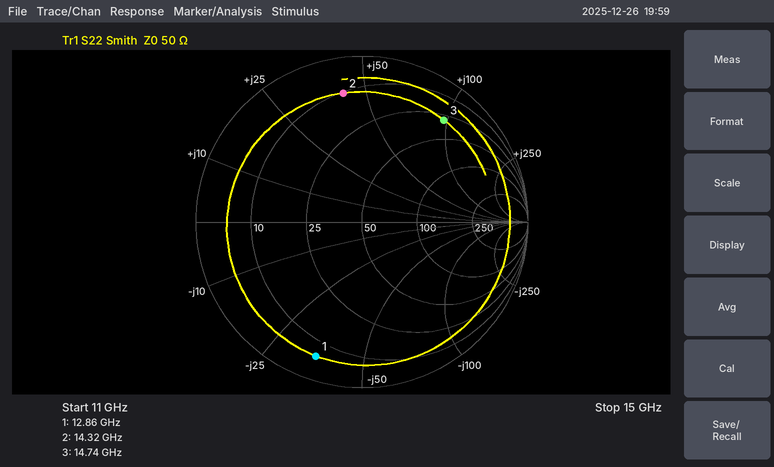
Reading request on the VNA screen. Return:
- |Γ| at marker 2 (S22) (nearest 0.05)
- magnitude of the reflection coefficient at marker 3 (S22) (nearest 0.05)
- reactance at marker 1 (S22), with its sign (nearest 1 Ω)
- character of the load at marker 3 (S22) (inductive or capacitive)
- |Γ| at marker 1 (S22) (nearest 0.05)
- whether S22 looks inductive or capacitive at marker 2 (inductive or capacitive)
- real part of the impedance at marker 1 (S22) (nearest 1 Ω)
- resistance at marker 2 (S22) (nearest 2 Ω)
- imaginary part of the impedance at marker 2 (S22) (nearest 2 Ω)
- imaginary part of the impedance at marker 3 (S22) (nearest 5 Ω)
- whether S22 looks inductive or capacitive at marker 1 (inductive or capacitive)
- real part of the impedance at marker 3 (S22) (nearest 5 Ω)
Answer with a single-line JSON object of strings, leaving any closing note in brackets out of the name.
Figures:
{"|Γ| at marker 2 (S22)": "0.80", "magnitude of the reflection coefficient at marker 3 (S22)": "0.80", "reactance at marker 1 (S22), with its sign": "-35 Ω", "character of the load at marker 3 (S22)": "inductive", "|Γ| at marker 1 (S22)": "0.85", "whether S22 looks inductive or capacitive at marker 2": "inductive", "real part of the impedance at marker 1 (S22)": "6 Ω", "resistance at marker 2 (S22)": "10 Ω", "imaginary part of the impedance at marker 2 (S22)": "+42 Ω", "imaginary part of the impedance at marker 3 (S22)": "+95 Ω", "whether S22 looks inductive or capacitive at marker 1": "capacitive", "real part of the impedance at marker 3 (S22)": "30 Ω"}
